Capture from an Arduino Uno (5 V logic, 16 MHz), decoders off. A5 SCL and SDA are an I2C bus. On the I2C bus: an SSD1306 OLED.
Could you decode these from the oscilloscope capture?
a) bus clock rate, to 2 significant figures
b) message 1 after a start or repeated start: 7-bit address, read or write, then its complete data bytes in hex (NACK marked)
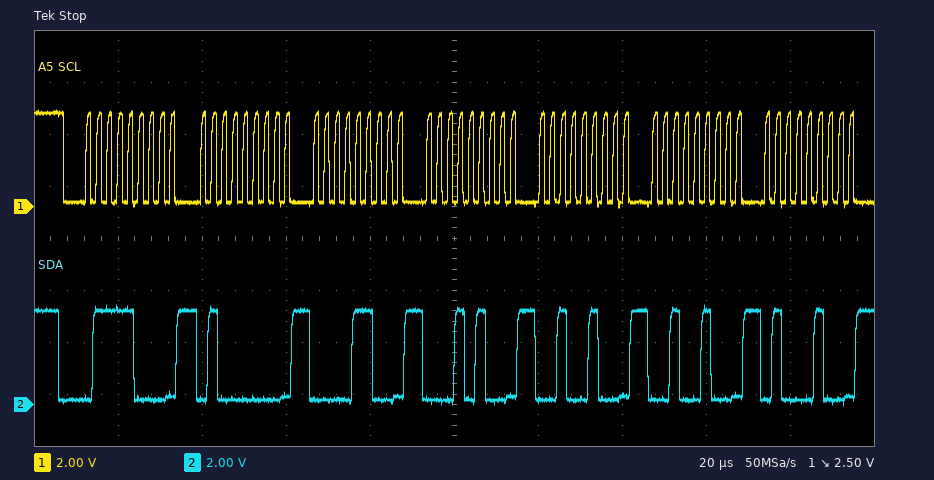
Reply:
400 kHz
0x3C write: 40 0C 14 24 24 44
